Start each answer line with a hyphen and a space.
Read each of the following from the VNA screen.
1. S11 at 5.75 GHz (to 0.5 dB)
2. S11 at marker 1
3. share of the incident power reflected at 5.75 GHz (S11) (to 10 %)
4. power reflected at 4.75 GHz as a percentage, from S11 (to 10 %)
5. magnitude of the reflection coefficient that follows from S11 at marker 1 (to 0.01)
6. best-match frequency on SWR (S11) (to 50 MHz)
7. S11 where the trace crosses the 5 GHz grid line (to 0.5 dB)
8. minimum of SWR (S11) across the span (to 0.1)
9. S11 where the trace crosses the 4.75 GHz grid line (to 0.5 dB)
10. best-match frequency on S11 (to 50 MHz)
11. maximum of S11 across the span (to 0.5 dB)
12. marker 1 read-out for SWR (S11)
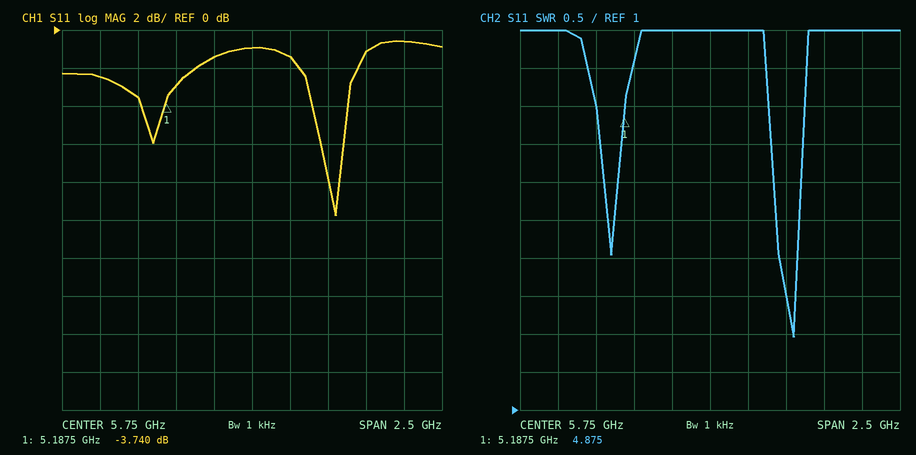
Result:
- -1.0 dB
- -3.740 dB
- 80 %
- 60 %
- 0.65
- 6.30 GHz
- -3.5 dB
- 2.0
- -2.5 dB
- 6.30 GHz
- -0.5 dB
- 4.875
